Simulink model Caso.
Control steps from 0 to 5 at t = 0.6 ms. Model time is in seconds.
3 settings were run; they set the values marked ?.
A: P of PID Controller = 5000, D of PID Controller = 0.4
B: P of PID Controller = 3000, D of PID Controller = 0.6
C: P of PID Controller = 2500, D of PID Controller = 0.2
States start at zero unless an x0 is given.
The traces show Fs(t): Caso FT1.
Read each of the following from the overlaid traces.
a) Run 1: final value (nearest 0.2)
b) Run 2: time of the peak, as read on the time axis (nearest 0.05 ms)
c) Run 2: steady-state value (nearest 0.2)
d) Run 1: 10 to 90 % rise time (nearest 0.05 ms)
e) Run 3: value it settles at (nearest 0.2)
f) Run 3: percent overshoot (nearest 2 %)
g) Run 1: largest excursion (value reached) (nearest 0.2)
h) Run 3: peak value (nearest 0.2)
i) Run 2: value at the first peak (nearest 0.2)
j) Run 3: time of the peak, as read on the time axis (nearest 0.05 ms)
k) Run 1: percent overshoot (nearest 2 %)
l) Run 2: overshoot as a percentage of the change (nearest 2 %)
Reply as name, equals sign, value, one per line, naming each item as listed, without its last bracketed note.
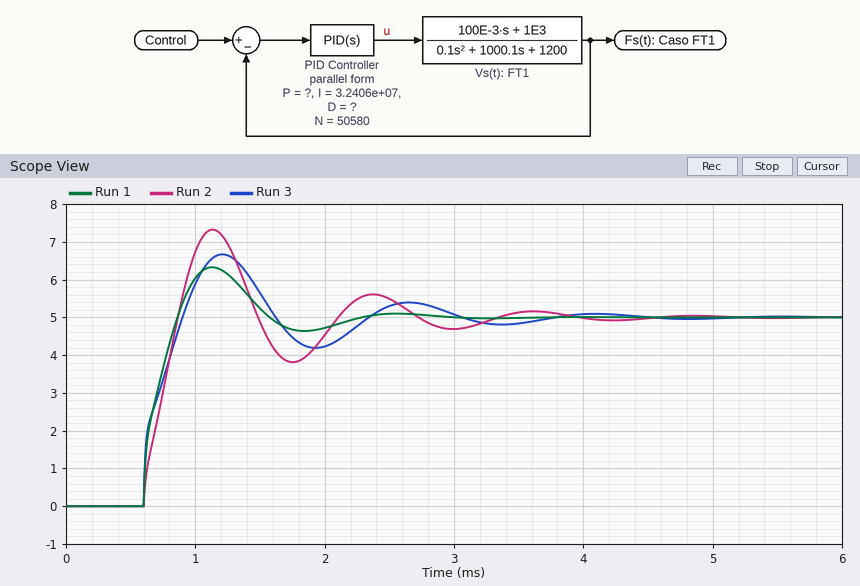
Run 1: final value = 5.0
Run 2: time of the peak, as read on the time axis = 1.15 ms
Run 2: steady-state value = 5.0
Run 1: 10 to 90 % rise time = 0.20 ms
Run 3: value it settles at = 5.0
Run 3: percent overshoot = 34 %
Run 1: largest excursion (value reached) = 6.4
Run 3: peak value = 6.6
Run 2: value at the first peak = 7.4
Run 3: time of the peak, as read on the time axis = 1.20 ms
Run 1: percent overshoot = 26 %
Run 2: overshoot as a percentage of the change = 46 %
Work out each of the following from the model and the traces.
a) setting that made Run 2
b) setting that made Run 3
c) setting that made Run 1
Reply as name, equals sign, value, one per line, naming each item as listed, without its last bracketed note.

setting that made Run 2 = C
setting that made Run 3 = B
setting that made Run 1 = A
